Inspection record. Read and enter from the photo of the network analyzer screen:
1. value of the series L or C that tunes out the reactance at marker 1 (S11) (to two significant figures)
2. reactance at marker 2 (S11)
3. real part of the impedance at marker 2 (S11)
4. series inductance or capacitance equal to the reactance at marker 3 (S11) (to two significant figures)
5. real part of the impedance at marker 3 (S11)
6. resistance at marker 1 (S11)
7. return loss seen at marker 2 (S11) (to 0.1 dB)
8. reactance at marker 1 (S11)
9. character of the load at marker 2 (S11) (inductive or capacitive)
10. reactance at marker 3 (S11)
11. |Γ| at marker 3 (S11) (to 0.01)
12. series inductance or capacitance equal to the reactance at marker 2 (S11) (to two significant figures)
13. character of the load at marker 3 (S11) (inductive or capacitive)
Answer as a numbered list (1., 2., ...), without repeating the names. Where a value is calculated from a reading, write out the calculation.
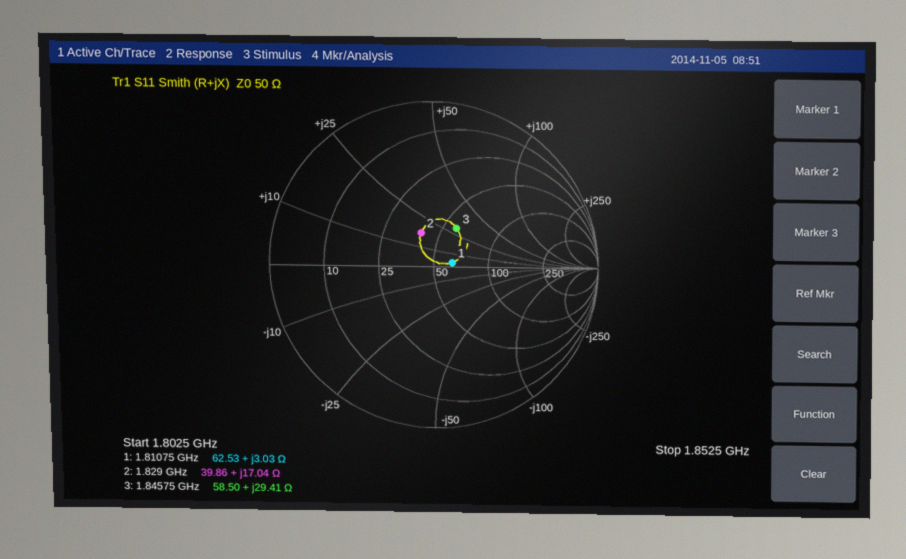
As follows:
1. C = 1/(2π × 1.81075 GHz × 3.03 Ω) ≈ 29 pF
2. +17.04 Ω
3. 39.86 Ω
4. L = 29.41 Ω/(2π × 1.84575 GHz) ≈ 2.5 nH
5. 58.50 Ω
6. 62.53 Ω
7. 13.3 dB
8. +3.03 Ω
9. inductive
10. +29.41 Ω
11. 0.27
12. L = 17.04 Ω/(2π × 1.829 GHz) ≈ 1.5 nH
13. inductive
